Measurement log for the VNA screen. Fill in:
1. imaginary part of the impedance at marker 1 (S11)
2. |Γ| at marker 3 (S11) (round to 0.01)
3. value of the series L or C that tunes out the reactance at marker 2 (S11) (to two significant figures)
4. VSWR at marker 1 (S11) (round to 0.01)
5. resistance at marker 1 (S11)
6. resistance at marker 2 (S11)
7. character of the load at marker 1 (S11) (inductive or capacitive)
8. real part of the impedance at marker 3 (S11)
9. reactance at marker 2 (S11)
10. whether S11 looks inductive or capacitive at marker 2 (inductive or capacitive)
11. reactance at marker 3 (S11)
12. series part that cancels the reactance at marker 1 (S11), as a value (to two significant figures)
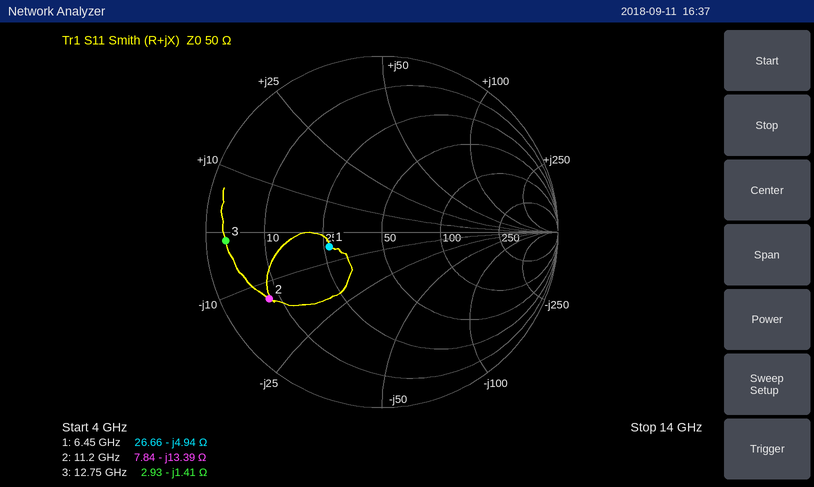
-4.94 Ω
0.89
190 pH
1.90
26.66 Ω
7.84 Ω
capacitive
2.93 Ω
-13.39 Ω
capacitive
-1.41 Ω
120 pH
